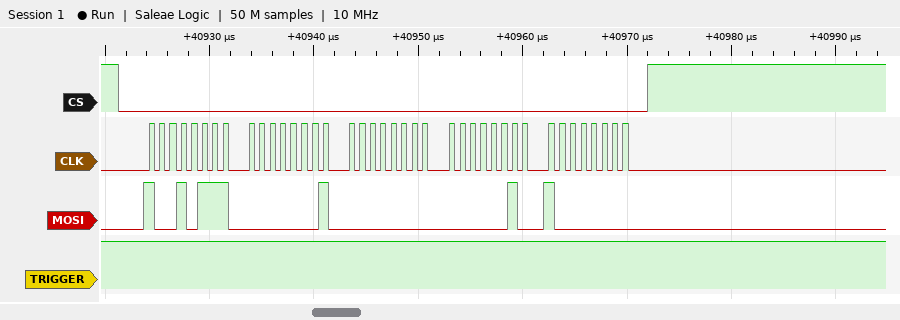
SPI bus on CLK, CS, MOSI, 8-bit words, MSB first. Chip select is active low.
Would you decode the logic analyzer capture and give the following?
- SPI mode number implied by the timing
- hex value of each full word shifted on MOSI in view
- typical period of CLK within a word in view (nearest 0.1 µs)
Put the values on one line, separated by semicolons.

0; 97, 01, 00, 02, 80; 1 µs
